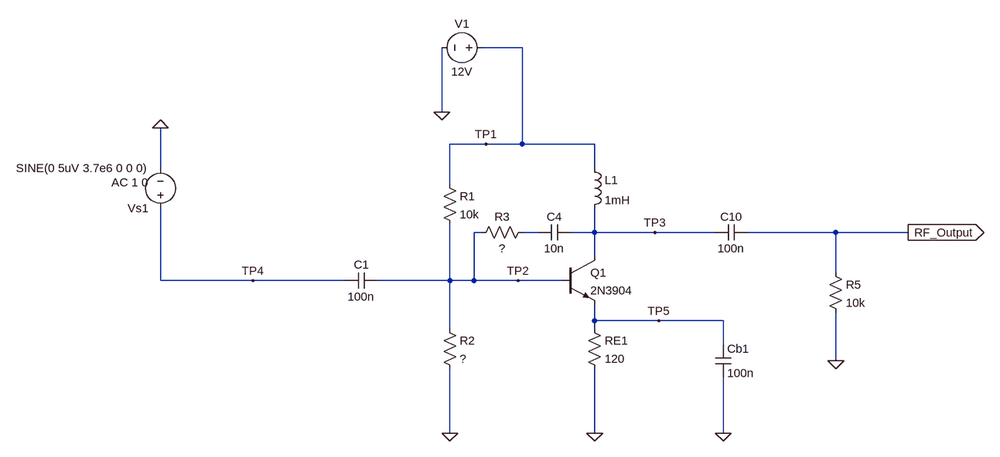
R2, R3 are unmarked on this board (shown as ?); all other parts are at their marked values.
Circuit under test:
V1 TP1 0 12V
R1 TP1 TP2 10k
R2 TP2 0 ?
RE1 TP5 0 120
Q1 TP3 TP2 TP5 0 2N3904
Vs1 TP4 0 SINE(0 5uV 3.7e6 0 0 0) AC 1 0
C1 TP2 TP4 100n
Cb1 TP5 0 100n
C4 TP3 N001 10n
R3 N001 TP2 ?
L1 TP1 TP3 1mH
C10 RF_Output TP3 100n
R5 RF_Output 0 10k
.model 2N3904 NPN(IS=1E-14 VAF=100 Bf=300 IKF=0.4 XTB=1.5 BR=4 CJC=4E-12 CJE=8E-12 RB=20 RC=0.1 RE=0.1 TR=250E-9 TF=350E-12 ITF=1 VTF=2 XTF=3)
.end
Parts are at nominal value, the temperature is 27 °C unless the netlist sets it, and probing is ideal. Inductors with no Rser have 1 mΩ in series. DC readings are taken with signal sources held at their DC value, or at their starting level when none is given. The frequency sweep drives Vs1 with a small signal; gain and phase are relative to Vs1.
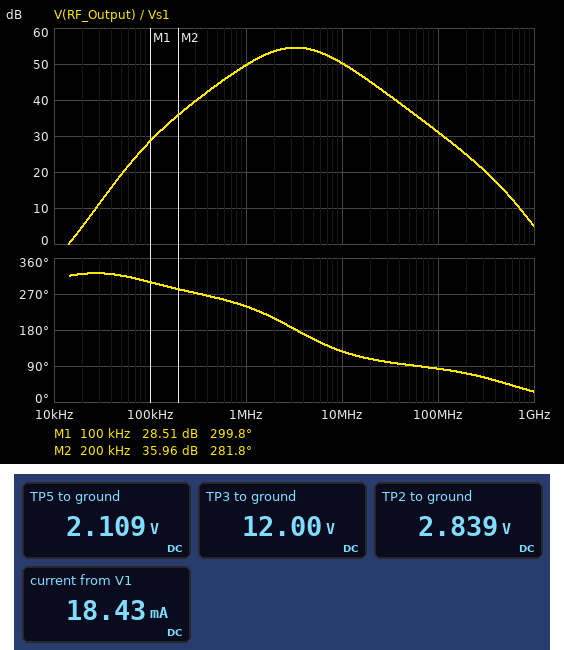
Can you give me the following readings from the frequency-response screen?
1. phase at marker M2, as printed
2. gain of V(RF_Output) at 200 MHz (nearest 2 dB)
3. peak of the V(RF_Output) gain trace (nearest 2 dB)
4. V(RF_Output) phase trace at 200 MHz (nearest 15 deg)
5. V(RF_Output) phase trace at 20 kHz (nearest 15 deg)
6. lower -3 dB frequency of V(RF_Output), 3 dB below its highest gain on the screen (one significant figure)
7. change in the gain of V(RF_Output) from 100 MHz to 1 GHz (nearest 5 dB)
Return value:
281.8 deg
24 dB
54 dB
75 deg
315 deg
1 MHz
-25 dB
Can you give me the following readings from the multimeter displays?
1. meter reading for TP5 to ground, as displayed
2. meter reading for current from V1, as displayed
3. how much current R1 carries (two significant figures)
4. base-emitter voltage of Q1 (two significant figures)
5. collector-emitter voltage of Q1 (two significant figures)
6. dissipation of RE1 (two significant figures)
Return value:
2.109 V
18.43 mA
920 µA
730 mV
9.9 V
37 mW
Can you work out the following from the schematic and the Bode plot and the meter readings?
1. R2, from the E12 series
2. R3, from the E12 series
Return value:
3.3 kΩ
1.2 kΩ
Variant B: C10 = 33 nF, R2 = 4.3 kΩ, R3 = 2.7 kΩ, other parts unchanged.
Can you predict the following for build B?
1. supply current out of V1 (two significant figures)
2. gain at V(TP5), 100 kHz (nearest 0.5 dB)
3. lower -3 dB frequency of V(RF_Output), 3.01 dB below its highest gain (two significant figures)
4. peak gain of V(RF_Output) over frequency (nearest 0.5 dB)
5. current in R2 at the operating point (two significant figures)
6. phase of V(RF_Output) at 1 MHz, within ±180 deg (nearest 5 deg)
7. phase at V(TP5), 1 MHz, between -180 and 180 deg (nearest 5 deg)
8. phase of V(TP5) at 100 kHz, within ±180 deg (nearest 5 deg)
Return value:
23 mA
-1.0 dB
1.2 MHz
60.5 dB
790 µA
-120 deg
-45 deg
-15 deg
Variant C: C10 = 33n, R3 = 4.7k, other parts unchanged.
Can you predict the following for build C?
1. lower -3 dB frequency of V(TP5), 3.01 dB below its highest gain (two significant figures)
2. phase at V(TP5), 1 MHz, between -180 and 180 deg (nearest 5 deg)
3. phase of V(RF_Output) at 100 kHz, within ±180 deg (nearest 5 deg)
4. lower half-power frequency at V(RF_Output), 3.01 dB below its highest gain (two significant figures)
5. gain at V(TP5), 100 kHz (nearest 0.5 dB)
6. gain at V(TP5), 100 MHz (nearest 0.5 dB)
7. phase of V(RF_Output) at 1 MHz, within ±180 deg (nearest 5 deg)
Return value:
750 Hz
-60 deg
-30 deg
950 kHz
-0.5 dB
-62.5 dB
-125 deg
